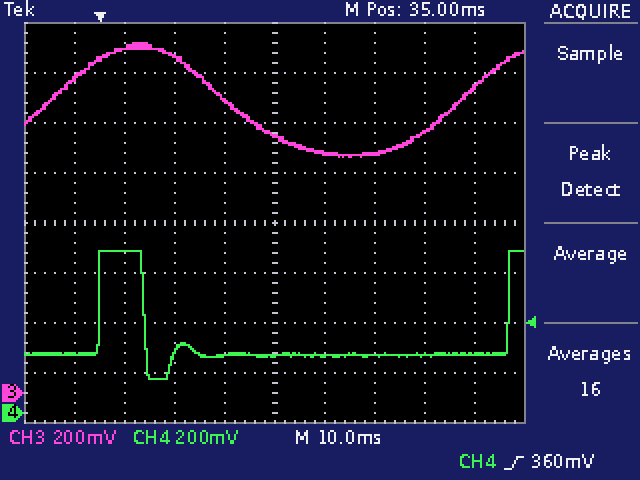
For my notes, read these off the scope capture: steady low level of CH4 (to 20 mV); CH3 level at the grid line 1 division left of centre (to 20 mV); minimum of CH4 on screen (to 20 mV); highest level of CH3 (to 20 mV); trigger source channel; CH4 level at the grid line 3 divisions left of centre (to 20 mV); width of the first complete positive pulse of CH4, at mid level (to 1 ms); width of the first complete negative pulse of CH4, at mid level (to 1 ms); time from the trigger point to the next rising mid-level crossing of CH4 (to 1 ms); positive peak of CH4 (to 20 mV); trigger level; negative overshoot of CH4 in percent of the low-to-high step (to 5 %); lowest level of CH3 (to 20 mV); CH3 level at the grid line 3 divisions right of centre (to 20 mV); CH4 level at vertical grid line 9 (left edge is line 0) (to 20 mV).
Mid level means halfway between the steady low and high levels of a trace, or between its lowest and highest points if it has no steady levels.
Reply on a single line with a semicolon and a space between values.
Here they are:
240 mV; 1.18 V; 140 mV; 1.40 V; CH4; 640 mV; 9 ms; 73 ms; 82 ms; 640 mV; 360 mV; 25 %; 940 mV; 1.04 V; 240 mV
